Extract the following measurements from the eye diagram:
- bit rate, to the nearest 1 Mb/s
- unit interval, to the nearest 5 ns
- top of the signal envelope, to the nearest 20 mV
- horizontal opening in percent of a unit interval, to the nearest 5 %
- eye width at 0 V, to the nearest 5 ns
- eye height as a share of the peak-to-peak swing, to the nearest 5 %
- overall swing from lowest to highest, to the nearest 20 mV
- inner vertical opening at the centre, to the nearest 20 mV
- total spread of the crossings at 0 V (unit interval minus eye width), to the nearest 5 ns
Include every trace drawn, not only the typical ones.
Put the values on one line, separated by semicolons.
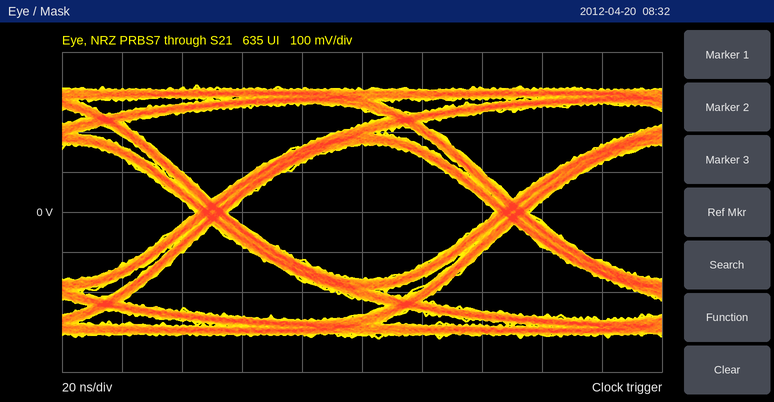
10 Mb/s; 100 ns; 320 mV; 90 %; 90 ns; 55 %; 640 mV; 340 mV; 10 ns
